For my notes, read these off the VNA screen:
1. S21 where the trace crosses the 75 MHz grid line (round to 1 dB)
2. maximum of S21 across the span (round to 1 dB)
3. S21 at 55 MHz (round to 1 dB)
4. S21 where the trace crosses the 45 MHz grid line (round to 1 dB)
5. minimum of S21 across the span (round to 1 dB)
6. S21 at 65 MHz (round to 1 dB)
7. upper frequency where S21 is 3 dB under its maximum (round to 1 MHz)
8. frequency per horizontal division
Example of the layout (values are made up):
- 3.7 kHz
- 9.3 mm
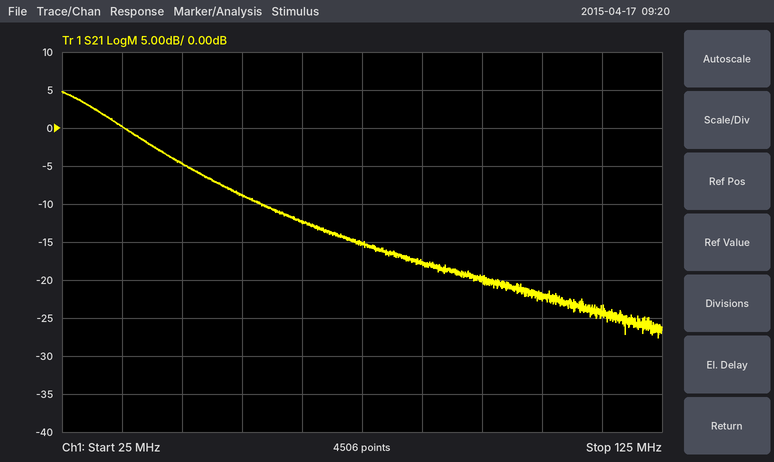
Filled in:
- -15 dB
- 5 dB
- -9 dB
- -5 dB
- -28 dB
- -12 dB
- 32 MHz
- 10 MHz
